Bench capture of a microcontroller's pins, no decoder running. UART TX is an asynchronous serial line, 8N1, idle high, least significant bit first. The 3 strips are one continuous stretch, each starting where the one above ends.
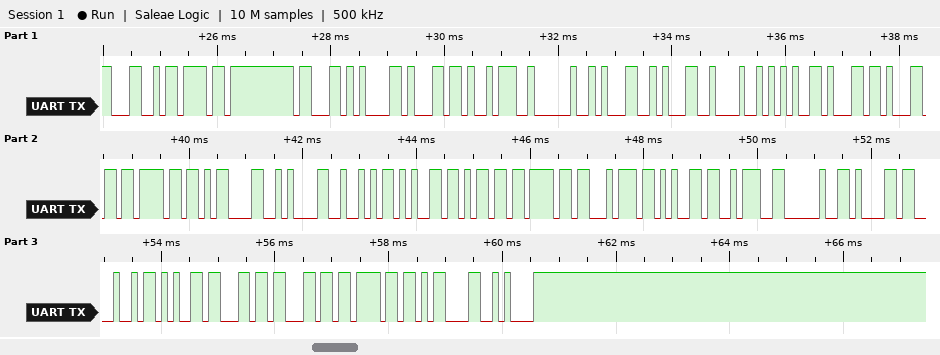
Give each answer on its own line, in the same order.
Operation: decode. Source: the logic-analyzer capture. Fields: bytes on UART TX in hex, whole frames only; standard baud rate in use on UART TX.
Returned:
4C 6F 63 61 6C 3A 20 31 31 48 65 6C 6C 6F 0D 0A 52 65 6D 6F 74 65 3A 20 61 48 65 6C 6C 6F 0D 0A
9600 baud
